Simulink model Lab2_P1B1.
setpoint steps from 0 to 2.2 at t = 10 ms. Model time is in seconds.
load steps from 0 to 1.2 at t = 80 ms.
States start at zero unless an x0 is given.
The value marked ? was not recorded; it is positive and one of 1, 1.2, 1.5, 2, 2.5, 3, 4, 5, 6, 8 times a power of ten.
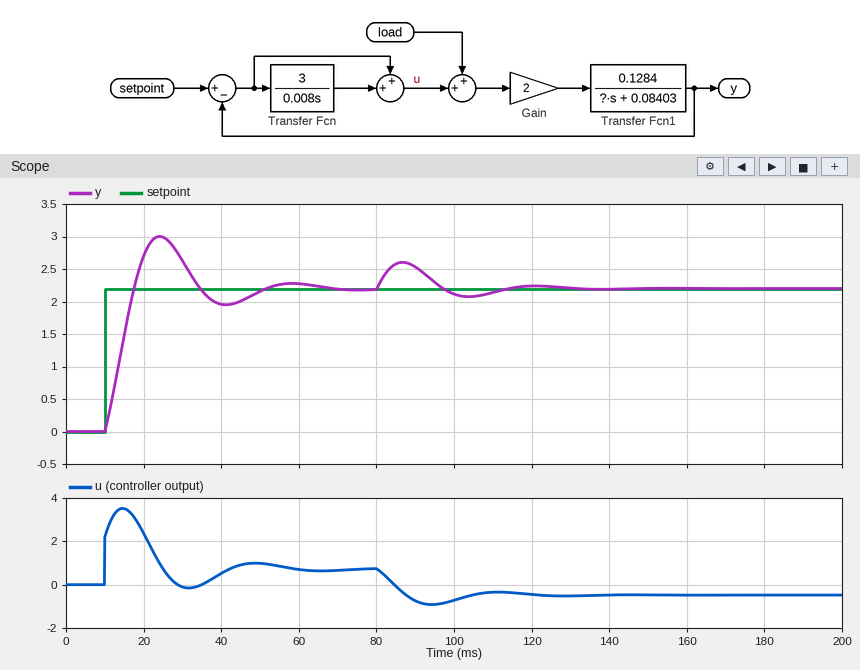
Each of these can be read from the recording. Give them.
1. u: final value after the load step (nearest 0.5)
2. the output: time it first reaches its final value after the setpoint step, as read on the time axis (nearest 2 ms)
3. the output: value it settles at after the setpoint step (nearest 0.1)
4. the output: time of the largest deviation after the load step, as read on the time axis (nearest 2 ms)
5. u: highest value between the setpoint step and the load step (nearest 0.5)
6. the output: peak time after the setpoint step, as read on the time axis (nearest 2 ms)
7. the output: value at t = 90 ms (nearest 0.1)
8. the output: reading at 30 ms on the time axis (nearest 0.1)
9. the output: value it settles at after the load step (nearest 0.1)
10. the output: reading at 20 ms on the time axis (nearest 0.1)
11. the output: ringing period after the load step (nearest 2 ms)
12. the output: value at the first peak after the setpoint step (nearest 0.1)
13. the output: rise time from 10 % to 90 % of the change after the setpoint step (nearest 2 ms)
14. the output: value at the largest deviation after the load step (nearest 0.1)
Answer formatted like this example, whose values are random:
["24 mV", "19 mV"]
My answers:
["-0.5", "18 ms", "2.2", "86 ms", "3.5", "24 ms", "2.5", "2.6", "2.2", "2.7", "34 ms", "3.0", "6 ms", "2.6"]
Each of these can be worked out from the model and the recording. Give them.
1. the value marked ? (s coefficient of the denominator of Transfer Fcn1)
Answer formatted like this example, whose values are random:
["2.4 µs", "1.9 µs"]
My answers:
["0.0025"]
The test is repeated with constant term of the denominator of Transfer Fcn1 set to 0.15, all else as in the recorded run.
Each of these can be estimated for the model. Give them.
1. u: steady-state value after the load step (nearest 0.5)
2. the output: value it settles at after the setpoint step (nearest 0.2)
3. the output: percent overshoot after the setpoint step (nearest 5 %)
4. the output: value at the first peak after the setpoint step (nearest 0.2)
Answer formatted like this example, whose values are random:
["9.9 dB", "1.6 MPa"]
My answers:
["0.0", "2.2", "30 %", "2.8"]
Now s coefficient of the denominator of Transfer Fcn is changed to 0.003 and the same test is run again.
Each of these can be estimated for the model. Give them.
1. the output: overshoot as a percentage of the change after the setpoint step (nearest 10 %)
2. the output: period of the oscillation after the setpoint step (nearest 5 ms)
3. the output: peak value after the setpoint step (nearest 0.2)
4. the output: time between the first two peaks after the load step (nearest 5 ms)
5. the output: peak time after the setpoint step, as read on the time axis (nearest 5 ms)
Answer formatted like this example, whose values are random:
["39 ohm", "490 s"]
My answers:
["50 %", "20 ms", "3.4", "20 ms", "20 ms"]
